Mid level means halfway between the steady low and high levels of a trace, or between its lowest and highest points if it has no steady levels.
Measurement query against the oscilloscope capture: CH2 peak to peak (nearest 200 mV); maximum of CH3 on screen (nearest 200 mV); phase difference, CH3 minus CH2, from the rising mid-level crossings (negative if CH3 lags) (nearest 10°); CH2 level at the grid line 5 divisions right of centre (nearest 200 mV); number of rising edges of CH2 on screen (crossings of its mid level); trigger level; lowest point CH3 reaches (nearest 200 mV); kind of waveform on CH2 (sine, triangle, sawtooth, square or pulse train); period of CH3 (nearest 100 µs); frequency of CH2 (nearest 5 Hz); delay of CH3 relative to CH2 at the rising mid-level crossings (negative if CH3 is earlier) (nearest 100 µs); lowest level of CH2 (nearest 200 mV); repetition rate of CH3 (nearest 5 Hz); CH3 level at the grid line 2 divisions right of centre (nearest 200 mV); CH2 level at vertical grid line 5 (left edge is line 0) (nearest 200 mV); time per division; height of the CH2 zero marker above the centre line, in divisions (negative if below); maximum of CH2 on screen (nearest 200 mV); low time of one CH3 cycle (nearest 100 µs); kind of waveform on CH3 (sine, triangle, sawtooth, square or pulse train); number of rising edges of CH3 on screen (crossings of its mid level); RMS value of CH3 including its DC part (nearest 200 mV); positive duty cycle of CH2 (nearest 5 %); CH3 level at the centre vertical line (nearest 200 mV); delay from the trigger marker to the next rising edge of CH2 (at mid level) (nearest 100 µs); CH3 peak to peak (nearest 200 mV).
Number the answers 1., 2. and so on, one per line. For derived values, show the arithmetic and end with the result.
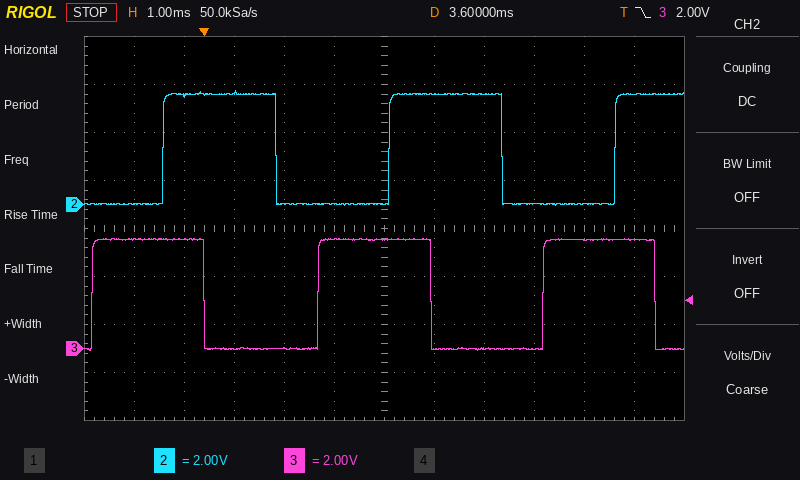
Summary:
1. 4.8 V − (0.0 V) = 4.8 V
2. 4.6 V
3. −360° × (-1.4 ms) / 4.5 ms ≈ +112°, so +110° to the nearest 10°
4. 4.6 V
5. 3
6. 2.00 V
7. 0.0 V
8. square
9. 4.5 ms
10. 1 / 4.5 ms ≈ 222 Hz, so 220 Hz to the nearest 5 Hz
11. -1.4 ms
12. 0.0 V
13. 1 / 4.5 ms ≈ 222 Hz, so 220 Hz to the nearest 5 Hz
14. 0.0 V
15. 0.0 V
16. 1 ms
17. +0.5 div
18. 4.8 V
19. 2.3 ms
20. square
21. 3
22. √(0.5 × (4.6 V)² + 0.5 × (0.0 V)²) ≈ 3.2 V
23. 50 %
24. 4.6 V
25. 3.7 ms
26. 4.6 V − (0.0 V) = 4.6 V
